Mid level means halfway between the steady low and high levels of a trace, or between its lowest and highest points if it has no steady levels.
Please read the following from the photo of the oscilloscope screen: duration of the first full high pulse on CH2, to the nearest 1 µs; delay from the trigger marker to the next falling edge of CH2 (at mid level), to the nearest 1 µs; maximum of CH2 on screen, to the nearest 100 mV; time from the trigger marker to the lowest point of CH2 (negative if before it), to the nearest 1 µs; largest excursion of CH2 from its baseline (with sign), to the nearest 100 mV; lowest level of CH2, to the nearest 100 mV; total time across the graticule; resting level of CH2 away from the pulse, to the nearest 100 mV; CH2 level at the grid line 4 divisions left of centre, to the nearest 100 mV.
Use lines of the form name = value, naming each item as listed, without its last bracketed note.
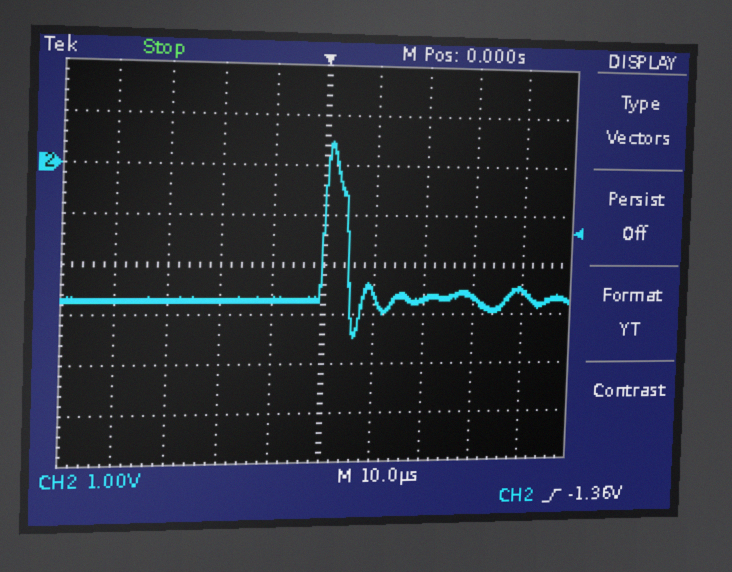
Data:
duration of the first full high pulse on CH2, to the nearest 1 µs = 5 µs
delay from the trigger marker to the next falling edge of CH2 (at mid level), to the nearest 1 µs = 5 µs
maximum of CH2 on screen, to the nearest 100 mV = 500 mV
time from the trigger marker to the lowest point of CH2 (negative if before it), to the nearest 1 µs = +6 µs
largest excursion of CH2 from its baseline (with sign), to the nearest 100 mV = +3.2 V
lowest level of CH2, to the nearest 100 mV = -3.5 V
total time across the graticule = 100 µs
resting level of CH2 away from the pulse, to the nearest 100 mV = -2.7 V
CH2 level at the grid line 4 divisions left of centre, to the nearest 100 mV = -2.7 V
